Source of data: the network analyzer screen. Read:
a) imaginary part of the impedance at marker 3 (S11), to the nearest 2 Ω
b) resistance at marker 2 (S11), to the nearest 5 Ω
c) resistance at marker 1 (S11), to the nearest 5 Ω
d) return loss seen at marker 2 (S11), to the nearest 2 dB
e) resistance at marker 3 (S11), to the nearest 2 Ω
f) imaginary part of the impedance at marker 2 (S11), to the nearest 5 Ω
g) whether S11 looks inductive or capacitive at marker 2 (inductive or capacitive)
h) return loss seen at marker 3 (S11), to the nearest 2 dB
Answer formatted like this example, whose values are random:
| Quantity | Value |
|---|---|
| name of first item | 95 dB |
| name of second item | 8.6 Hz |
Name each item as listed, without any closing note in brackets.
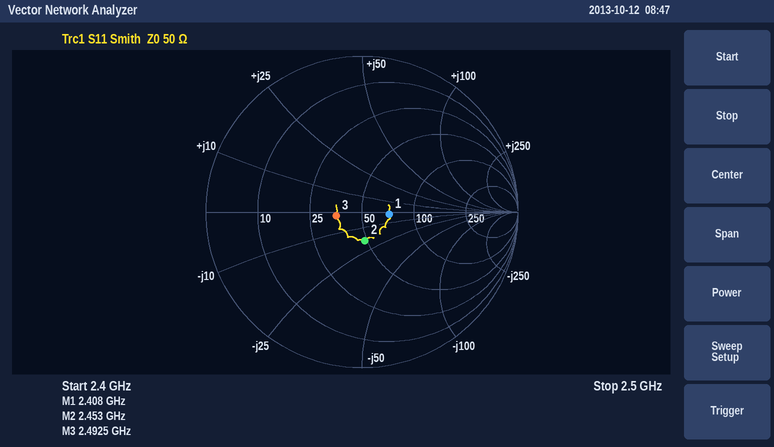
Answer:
| Quantity | Value |
|---|---|
| imaginary part of the impedance at marker 3 (S11), to the nearest 2 Ω | -2 Ω |
| resistance at marker 2 (S11), to the nearest 5 Ω | 50 Ω |
| resistance at marker 1 (S11), to the nearest 5 Ω | 70 Ω |
| return loss seen at marker 2 (S11), to the nearest 2 dB | 14 dB |
| resistance at marker 3 (S11), to the nearest 2 Ω | 36 Ω |
| imaginary part of the impedance at marker 2 (S11), to the nearest 5 Ω | -20 Ω |
| whether S11 looks inductive or capacitive at marker 2 | capacitive |
| return loss seen at marker 3 (S11), to the nearest 2 dB | 16 dB |
